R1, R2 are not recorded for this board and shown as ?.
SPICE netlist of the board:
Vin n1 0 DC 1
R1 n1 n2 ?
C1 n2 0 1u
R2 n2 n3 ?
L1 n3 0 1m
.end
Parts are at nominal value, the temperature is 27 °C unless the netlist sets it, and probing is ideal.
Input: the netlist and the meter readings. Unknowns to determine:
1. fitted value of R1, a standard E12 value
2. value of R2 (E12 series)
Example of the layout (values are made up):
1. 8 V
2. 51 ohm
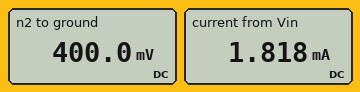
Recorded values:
1. 330 Ω
2. 220 Ω
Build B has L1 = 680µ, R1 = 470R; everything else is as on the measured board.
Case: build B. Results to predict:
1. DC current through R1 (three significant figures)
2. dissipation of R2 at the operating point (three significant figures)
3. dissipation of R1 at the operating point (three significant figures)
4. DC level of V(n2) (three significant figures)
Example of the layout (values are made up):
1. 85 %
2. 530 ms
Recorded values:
1. 1.45 mA
2. 462 µW
3. 987 µW
4. 319 mV
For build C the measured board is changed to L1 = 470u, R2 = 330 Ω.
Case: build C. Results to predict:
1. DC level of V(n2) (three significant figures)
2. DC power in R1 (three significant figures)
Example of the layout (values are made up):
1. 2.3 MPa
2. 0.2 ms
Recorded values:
1. 500 mV
2. 758 µW
